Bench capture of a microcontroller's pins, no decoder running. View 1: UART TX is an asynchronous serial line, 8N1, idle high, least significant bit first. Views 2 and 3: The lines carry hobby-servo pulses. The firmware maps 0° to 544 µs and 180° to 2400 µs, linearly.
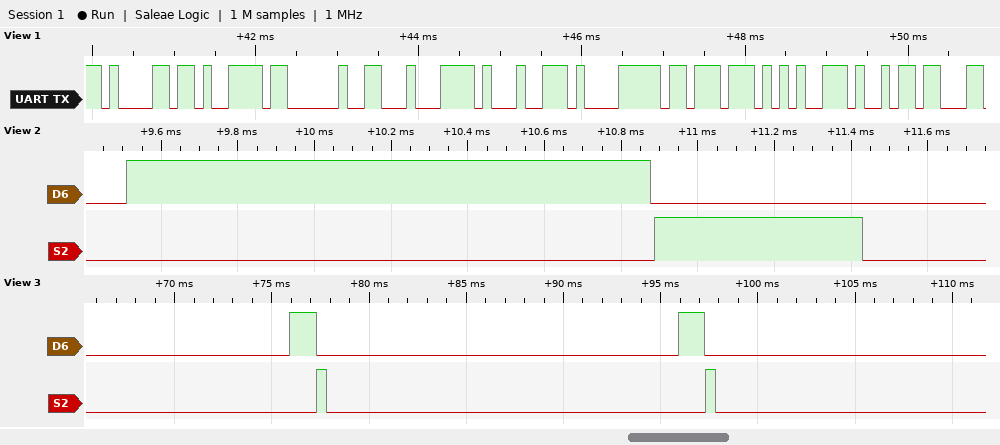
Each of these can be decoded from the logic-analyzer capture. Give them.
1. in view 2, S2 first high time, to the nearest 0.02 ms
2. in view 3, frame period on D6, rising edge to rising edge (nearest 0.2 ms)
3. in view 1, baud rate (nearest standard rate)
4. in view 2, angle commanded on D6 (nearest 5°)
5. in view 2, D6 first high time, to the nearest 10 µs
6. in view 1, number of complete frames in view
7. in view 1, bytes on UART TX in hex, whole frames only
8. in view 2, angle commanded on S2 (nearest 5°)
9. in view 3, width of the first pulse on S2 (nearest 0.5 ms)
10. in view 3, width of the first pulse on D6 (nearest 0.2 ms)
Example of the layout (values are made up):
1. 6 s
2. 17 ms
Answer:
1. 0.54 ms
2. 20.0 ms
3. 9600 baud
4. 80°
5. 1370 µs
6. 9
7. 0x61 0x79 0x20 0xC4 0x91 0xE1 0xBB 0x95 0x69
8. 0°
9. 0.5 ms
10. 1.4 ms
